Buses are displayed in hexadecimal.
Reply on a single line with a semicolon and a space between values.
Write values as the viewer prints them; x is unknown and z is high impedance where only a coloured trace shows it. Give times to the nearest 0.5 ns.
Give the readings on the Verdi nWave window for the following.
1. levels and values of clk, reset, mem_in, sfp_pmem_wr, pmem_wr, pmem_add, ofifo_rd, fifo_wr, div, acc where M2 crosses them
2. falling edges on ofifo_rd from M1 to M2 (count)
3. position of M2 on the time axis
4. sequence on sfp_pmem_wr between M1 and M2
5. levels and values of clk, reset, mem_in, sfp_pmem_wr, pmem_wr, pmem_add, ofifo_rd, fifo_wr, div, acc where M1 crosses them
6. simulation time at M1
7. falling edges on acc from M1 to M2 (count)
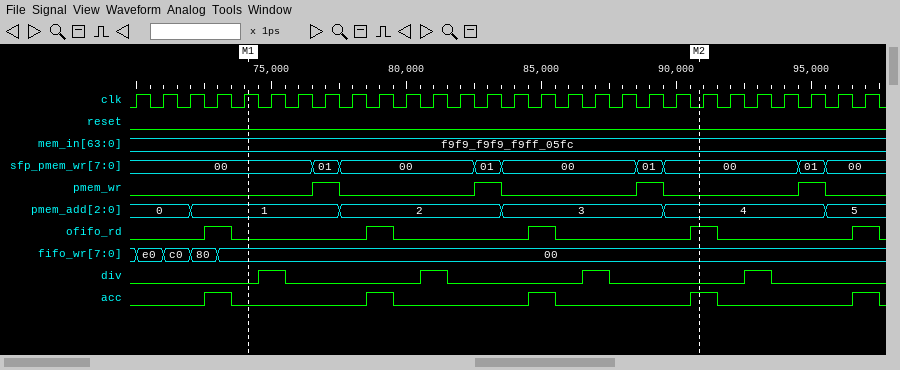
clk=0, reset=0, mem_in=f9f9_f9f9_f9ff_05fc, sfp_pmem_wr=00, pmem_wr=0, pmem_add=4, ofifo_rd=1, fifo_wr=00, div=0, acc=1; 2; 91 ns; 00, 01, 00, 01, 00, 01, 00; clk=1, reset=0, mem_in=f9f9_f9f9_f9ff_05fc, sfp_pmem_wr=00, pmem_wr=0, pmem_add=1, ofifo_rd=0, fifo_wr=00, div=0, acc=0; 74 ns; 2
